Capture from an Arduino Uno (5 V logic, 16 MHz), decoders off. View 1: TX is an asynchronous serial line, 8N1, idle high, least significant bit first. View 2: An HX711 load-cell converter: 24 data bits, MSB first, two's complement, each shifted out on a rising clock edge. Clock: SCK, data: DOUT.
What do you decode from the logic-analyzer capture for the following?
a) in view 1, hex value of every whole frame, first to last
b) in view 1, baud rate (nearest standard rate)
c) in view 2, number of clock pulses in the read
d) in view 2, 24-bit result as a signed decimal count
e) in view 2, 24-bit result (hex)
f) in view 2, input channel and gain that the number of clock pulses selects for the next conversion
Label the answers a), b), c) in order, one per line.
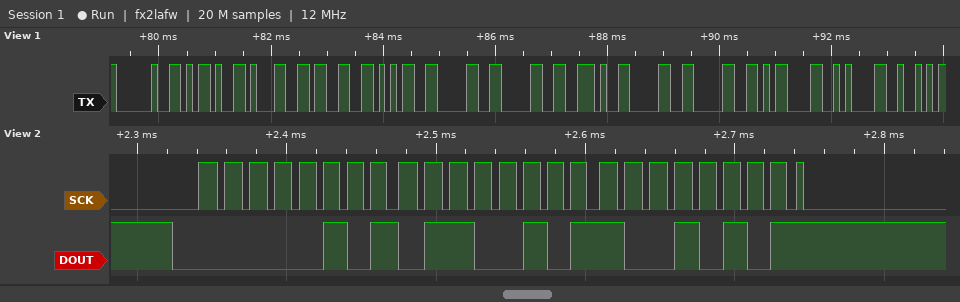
a) 0x20 0x2D 0x31 0x33 0x35 0x30 0x30 0x2E 0x30 0x30 0x0D 0x0A 0x52
b) 9600 baud
c) 25
d) 353685
e) 0x056595
f) channel A, gain 128
